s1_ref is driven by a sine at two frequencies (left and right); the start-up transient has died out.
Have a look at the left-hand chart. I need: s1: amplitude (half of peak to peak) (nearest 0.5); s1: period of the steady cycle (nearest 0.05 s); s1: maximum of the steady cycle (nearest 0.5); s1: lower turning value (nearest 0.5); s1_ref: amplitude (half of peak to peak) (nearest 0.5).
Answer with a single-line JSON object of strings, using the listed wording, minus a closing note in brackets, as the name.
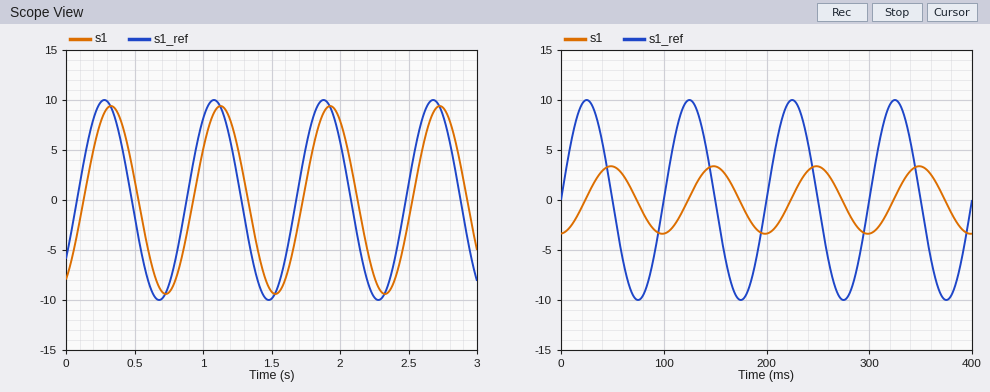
{"s1: amplitude (half of peak to peak)": "9.5", "s1: period of the steady cycle": "0.80 s", "s1: maximum of the steady cycle": "9.5", "s1: lower turning value": "-9.5", "s1_ref: amplitude (half of peak to peak)": "10.0"}
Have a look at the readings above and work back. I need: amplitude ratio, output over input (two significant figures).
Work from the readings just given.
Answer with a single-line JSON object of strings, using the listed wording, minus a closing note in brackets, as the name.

{"amplitude ratio, output over input": "0.95"}
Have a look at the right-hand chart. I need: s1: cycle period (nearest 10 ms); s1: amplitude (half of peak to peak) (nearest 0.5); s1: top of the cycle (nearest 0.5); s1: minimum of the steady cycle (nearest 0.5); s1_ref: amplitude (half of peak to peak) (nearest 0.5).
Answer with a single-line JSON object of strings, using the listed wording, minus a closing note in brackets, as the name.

{"s1: cycle period": "100 ms", "s1: amplitude (half of peak to peak)": "3.5", "s1: top of the cycle": "3.5", "s1: minimum of the steady cycle": "-3.5", "s1_ref: amplitude (half of peak to peak)": "10.0"}
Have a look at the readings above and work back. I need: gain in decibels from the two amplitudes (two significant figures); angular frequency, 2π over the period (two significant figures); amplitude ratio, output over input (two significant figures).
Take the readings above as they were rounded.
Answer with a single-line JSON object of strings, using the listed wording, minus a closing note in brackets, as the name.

{"gain in decibels from the two amplitudes": "-9.1 dB", "angular frequency, 2π over the period": "0.063 rad/ms", "amplitude ratio, output over input": "0.35"}
